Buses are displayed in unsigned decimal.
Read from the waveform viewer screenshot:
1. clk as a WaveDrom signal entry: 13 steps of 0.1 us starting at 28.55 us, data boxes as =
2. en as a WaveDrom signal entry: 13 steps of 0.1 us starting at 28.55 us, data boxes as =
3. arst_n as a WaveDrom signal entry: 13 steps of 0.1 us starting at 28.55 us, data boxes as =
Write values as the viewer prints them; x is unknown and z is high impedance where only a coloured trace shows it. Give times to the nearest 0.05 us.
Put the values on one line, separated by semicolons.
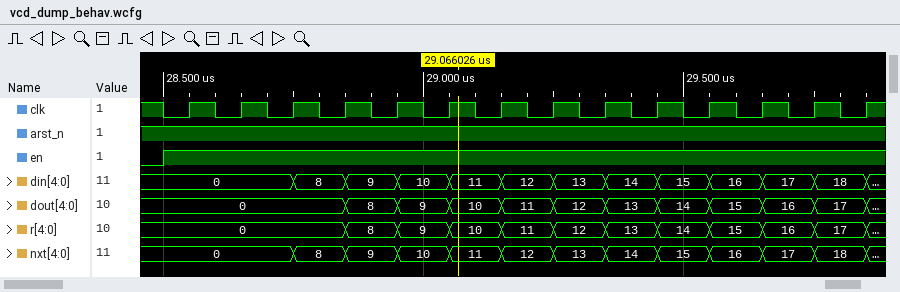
{name: 'clk', wave: 'p............'}; {name: 'en', wave: '1............'}; {name: 'arst_n', wave: '1............'}
